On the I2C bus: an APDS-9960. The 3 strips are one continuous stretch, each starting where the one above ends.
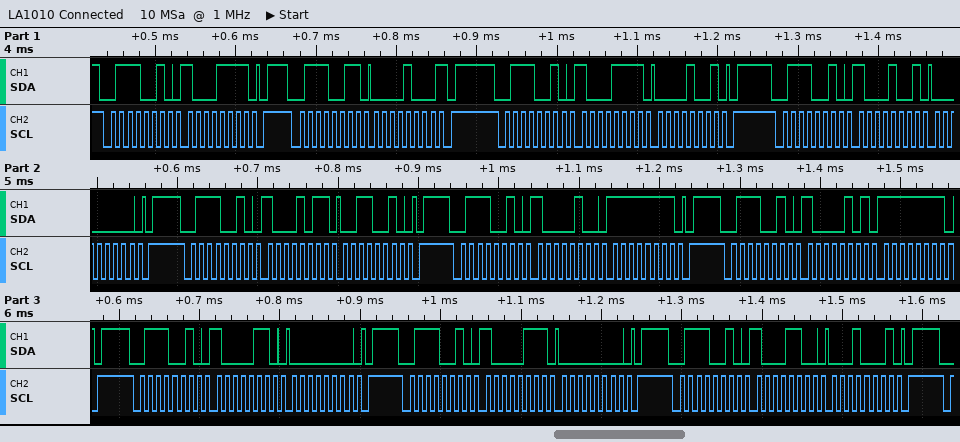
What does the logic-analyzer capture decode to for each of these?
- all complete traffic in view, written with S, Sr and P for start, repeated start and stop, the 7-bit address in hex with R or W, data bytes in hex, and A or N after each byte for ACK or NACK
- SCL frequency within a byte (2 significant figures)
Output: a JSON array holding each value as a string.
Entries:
["S 39W A 8F A P S 39R A 08 N P S 39W A 8F A 09 A P S 39W A 89 A 00 A P S 39W A 8B A 32 A P S 39W A 84 A FF A P S 39W A 85 A FF A P S 39W A 86 A 00 A P S 39W A 87 A 00 A P S 39W A 8C A 11 A P", "100 kHz"]
